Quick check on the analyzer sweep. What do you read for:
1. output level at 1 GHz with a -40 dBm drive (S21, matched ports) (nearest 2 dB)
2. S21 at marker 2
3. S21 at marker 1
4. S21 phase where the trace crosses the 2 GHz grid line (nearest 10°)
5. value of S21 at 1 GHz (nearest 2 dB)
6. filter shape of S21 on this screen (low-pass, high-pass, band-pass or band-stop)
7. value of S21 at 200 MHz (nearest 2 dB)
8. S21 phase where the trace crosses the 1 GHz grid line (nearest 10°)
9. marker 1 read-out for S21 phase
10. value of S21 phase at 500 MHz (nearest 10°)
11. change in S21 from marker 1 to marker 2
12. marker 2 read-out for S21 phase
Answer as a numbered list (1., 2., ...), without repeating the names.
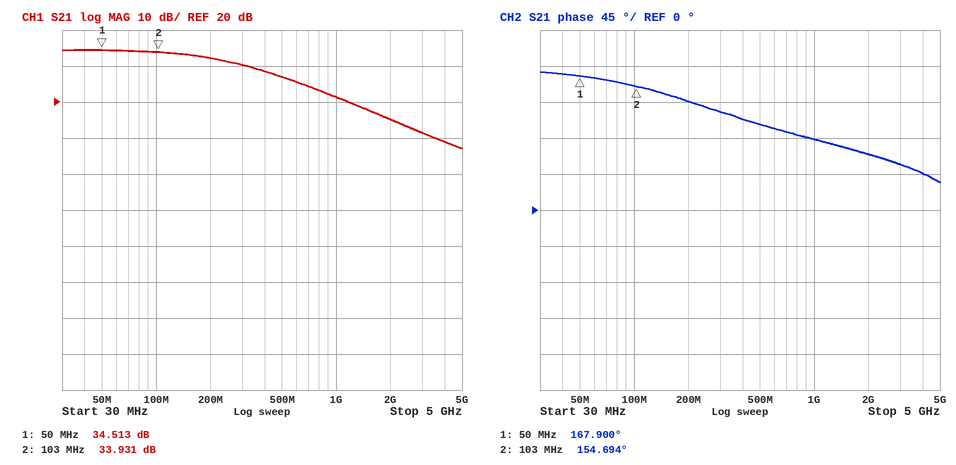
1. -18 dBm
2. 33.931 dB
3. 34.513 dB
4. 70°
5. 22 dB
6. low-pass
7. 32 dB
8. 90°
9. 167.900°
10. 110°
11. -0.582 dB
12. 154.694°
